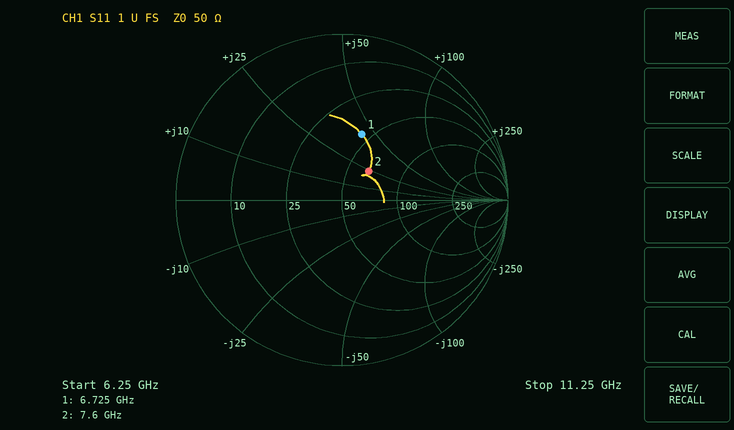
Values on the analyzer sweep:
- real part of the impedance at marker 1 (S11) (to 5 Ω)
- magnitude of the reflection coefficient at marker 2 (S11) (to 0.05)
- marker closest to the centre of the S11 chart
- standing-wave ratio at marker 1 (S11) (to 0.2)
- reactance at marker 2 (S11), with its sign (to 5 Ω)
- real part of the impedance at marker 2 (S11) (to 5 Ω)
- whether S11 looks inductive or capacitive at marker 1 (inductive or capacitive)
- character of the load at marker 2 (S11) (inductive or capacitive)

45 Ω
0.25
marker 2
2.4
+25 Ω
65 Ω
inductive
inductive
